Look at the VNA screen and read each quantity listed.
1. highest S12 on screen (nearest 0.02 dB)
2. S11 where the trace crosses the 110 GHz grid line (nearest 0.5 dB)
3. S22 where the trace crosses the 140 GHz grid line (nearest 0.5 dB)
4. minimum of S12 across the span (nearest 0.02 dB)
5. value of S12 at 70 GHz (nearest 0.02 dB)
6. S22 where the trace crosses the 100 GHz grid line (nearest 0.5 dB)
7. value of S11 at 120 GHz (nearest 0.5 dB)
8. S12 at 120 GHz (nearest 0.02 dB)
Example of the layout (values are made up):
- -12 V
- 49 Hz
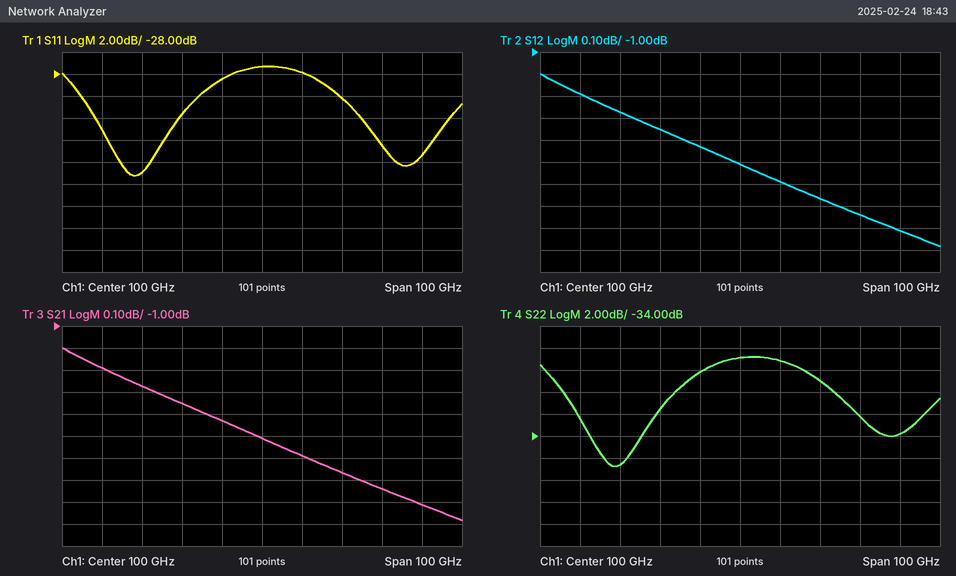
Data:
- -1.10 dB
- -28.0 dB
- -34.0 dB
- -1.88 dB
- -1.28 dB
- -27.0 dB
- -30.0 dB
- -1.66 dB
